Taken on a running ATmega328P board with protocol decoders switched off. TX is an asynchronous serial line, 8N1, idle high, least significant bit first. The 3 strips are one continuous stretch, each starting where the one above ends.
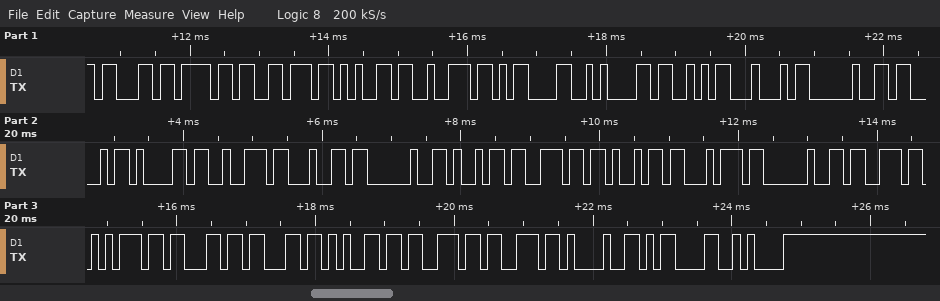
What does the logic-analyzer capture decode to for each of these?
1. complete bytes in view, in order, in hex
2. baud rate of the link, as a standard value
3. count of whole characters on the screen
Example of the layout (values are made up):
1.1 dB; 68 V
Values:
63 6F 76 65 72 0D 0A 53 44 20 43 61 72 64 20 69 6E 69 74 20 73 75 63 63 65 73 73 21 0D 0A; 9600 baud; 30
